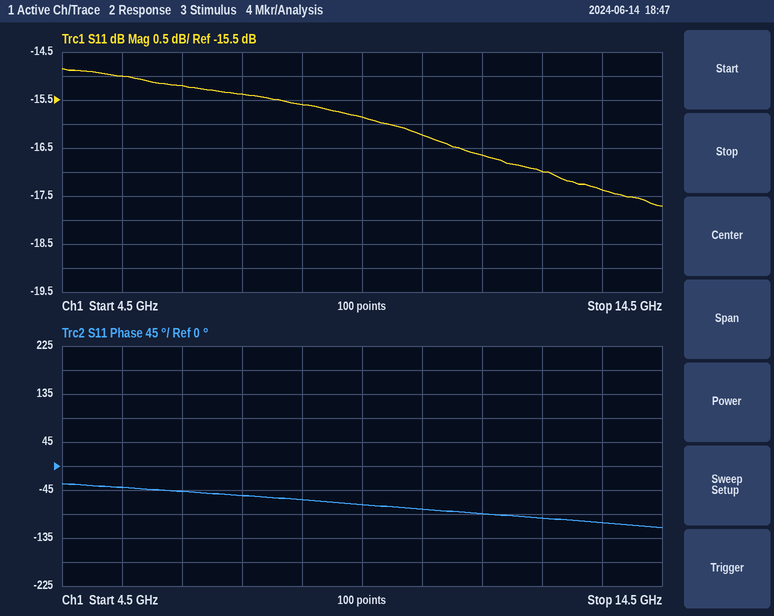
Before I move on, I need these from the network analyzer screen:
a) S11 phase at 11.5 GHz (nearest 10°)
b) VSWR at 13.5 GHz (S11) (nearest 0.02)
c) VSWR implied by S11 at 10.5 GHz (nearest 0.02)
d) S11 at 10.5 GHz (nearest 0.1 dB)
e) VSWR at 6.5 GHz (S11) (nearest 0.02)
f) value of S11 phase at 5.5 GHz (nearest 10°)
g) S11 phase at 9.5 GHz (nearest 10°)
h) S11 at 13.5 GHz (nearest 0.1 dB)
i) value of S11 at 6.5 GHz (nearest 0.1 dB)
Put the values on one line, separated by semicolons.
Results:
-90°; 1.32; 1.36; -16.2 dB; 1.42; -40°; -70°; -17.4 dB; -15.2 dB
